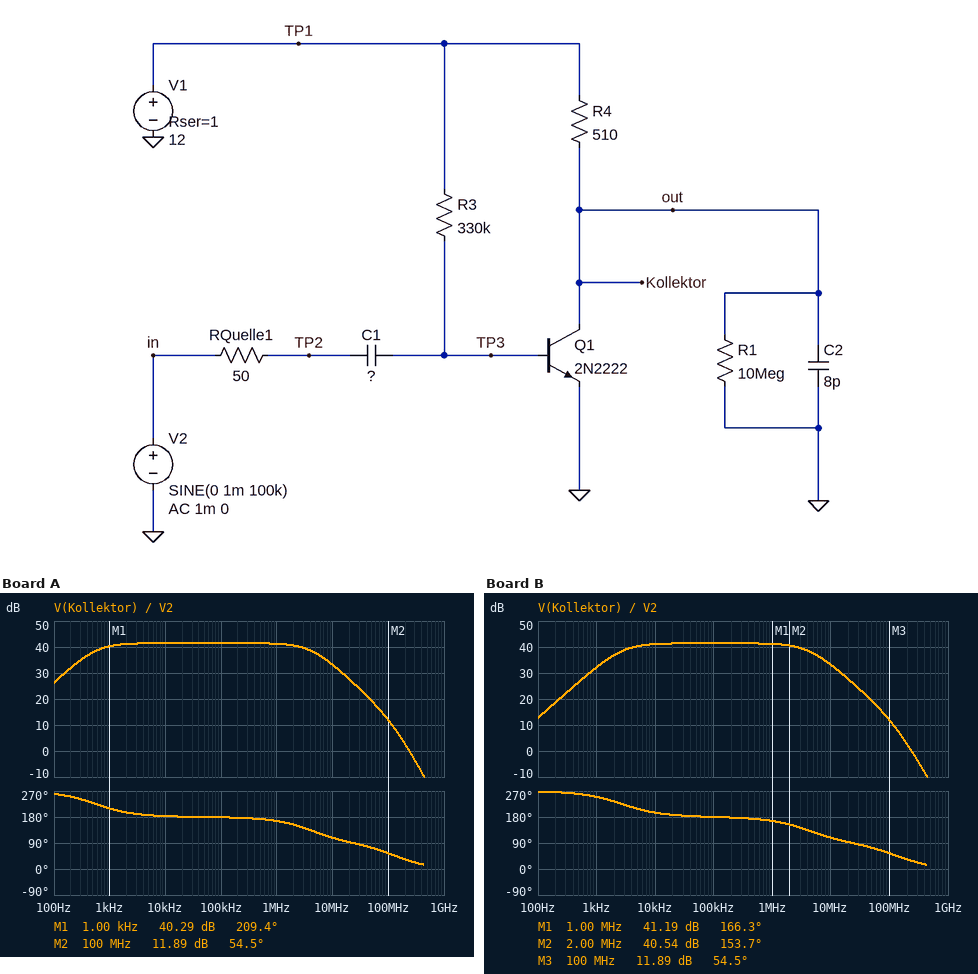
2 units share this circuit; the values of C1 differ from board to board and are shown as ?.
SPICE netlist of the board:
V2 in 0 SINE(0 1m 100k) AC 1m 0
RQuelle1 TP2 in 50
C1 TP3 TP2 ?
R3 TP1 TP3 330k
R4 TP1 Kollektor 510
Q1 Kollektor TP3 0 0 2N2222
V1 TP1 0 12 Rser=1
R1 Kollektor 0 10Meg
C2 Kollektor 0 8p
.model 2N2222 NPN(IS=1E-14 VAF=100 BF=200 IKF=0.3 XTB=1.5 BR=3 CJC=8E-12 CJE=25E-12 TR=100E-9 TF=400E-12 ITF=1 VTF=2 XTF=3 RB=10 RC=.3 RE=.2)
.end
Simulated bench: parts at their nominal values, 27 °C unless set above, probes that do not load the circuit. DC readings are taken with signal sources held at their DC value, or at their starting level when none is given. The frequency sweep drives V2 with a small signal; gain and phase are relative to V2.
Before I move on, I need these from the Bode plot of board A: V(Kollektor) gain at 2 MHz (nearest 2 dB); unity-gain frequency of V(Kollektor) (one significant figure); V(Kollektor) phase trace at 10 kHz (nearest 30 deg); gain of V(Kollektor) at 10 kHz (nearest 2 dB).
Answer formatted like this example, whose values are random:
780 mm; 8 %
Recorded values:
40 dB; 200 MHz; 180 deg; 42 dB
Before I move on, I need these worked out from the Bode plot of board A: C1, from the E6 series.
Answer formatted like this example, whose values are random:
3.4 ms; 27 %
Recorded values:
330 nF
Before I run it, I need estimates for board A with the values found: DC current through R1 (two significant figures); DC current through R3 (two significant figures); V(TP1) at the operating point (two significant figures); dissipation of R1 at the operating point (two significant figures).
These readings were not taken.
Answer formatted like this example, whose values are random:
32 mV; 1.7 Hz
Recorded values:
830 nA; 34 µA; 12 V; 6.9 µW
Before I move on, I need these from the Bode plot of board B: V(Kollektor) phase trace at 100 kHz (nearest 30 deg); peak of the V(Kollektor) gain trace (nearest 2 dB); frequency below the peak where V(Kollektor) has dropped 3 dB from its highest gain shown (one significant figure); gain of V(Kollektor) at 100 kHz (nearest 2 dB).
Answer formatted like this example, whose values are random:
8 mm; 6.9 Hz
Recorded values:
180 deg; 42 dB; 3 kHz; 42 dB
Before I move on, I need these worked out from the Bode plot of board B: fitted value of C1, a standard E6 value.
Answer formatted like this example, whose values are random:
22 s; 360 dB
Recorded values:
68 nF
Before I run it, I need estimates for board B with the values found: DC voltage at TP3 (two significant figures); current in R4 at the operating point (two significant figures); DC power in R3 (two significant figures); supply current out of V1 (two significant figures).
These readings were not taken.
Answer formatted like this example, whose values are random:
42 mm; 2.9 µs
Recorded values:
710 mV; 7.2 mA; 390 µW; 7.2 mA
